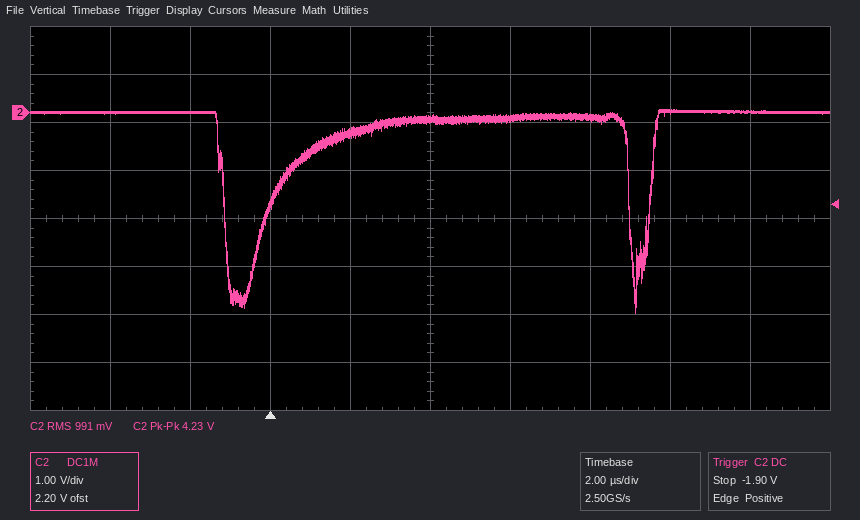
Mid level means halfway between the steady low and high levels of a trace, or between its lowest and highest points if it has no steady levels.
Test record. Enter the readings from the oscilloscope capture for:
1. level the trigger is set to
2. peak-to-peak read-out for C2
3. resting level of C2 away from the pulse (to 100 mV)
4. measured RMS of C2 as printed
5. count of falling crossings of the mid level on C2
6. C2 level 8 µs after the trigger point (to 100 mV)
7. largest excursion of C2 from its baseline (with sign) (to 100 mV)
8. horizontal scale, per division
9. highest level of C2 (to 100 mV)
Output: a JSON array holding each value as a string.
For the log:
["-1.90 V", "4.23 V", "0.0 V", "991 mV", "2", "-100 mV", "-4.2 V", "2 µs", "100 mV"]
